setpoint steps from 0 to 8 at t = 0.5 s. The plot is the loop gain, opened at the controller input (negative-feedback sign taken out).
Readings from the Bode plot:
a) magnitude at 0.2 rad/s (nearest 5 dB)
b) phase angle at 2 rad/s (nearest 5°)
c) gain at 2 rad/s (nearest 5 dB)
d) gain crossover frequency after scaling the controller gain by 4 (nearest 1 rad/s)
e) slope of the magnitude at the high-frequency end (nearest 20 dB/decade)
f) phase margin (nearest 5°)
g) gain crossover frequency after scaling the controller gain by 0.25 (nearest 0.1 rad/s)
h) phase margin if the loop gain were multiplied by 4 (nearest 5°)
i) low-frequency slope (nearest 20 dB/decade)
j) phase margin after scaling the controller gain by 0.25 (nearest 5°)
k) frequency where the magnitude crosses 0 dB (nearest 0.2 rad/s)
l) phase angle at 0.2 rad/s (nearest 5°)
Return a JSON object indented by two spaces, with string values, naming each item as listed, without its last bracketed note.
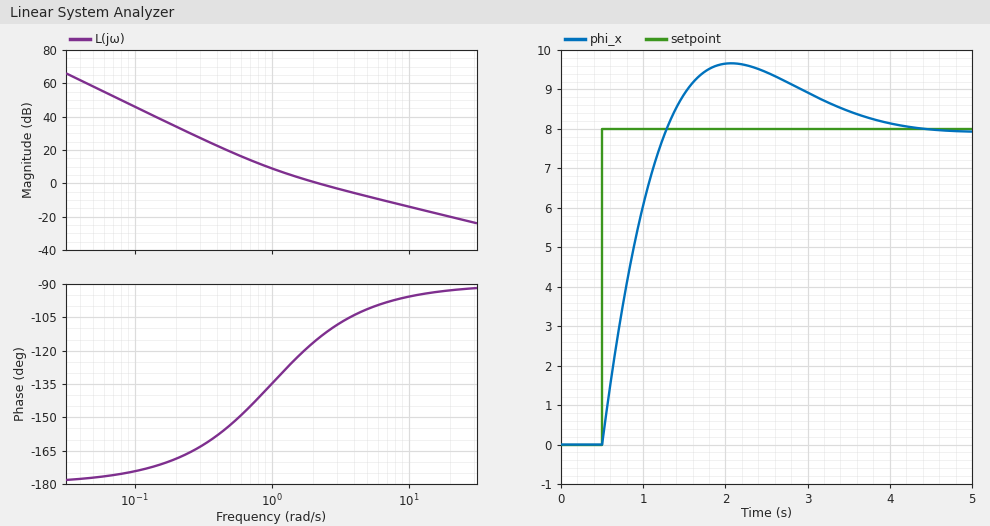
{
  "magnitude at 0.2 rad/s": "35 dB",
  "phase angle at 2 rad/s": "-115°",
  "gain at 2 rad/s": "0 dB",
  "gain crossover frequency after scaling the controller gain by 4": "8 rad/s",
  "slope of the magnitude at the high-frequency end": "-20 dB/decade",
  "phase margin": "65°",
  "gain crossover frequency after scaling the controller gain by 0.25": "0.8 rad/s",
  "phase margin if the loop gain were multiplied by 4": "85°",
  "low-frequency slope": "-40 dB/decade",
  "phase margin after scaling the controller gain by 0.25": "40°",
  "frequency where the magnitude crosses 0 dB": "2.2 rad/s",
  "phase angle at 0.2 rad/s": "-170°"
}
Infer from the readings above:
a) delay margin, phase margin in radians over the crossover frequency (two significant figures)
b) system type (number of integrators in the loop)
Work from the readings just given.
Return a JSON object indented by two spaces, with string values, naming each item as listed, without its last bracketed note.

{
  "delay margin, phase margin in radians over the crossover frequency": "0.52 s",
  "system type": "2"
}
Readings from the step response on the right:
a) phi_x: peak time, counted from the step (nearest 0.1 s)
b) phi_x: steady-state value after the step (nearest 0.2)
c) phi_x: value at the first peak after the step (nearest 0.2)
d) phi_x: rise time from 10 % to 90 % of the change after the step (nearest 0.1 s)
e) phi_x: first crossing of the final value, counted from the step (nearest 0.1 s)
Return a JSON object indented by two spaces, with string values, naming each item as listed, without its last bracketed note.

{
  "phi_x: peak time, counted from the step": "1.6 s",
  "phi_x: steady-state value after the step": "8.0",
  "phi_x: value at the first peak after the step": "9.6",
  "phi_x: rise time from 10 % to 90 % of the change after the step": "0.6 s",
  "phi_x: first crossing of the final value, counted from the step": "0.8 s"
}
